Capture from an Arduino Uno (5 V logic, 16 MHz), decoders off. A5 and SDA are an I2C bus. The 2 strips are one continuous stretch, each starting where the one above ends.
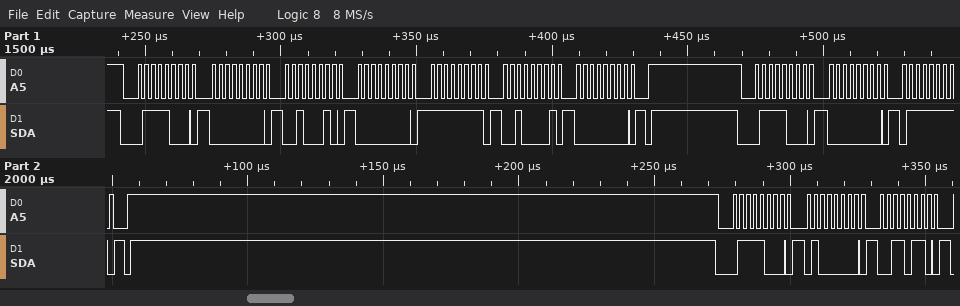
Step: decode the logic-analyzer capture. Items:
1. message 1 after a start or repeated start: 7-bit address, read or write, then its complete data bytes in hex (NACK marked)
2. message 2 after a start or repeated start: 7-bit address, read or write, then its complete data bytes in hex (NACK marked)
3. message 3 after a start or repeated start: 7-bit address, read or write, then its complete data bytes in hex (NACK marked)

0x3C write: 00 22 00 FF 21 00
0x3C write: 00 7F
0x3C write: 40 36
